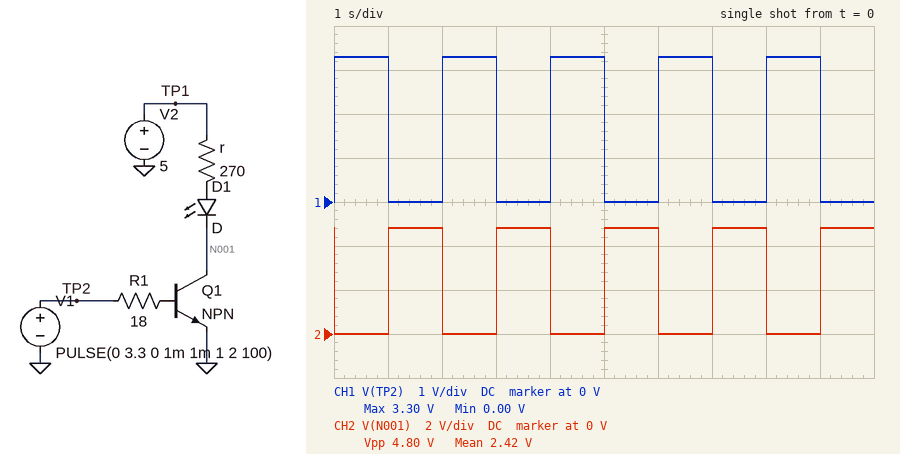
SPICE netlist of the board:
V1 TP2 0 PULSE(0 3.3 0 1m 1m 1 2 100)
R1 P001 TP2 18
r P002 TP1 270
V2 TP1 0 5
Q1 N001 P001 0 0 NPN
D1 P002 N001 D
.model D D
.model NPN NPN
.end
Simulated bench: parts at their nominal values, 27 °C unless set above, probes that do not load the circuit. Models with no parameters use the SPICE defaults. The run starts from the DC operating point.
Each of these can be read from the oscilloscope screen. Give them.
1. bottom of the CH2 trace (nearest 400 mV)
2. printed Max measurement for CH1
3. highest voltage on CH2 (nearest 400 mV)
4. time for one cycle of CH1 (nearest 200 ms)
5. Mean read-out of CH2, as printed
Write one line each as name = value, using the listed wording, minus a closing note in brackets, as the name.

bottom of the CH2 trace = 0 V
printed Max measurement for CH1 = 3.30 V
highest voltage on CH2 = 4.8 V
time for one cycle of CH1 = 2.0 s
Mean read-out of CH2, as printed = 2.42 V
